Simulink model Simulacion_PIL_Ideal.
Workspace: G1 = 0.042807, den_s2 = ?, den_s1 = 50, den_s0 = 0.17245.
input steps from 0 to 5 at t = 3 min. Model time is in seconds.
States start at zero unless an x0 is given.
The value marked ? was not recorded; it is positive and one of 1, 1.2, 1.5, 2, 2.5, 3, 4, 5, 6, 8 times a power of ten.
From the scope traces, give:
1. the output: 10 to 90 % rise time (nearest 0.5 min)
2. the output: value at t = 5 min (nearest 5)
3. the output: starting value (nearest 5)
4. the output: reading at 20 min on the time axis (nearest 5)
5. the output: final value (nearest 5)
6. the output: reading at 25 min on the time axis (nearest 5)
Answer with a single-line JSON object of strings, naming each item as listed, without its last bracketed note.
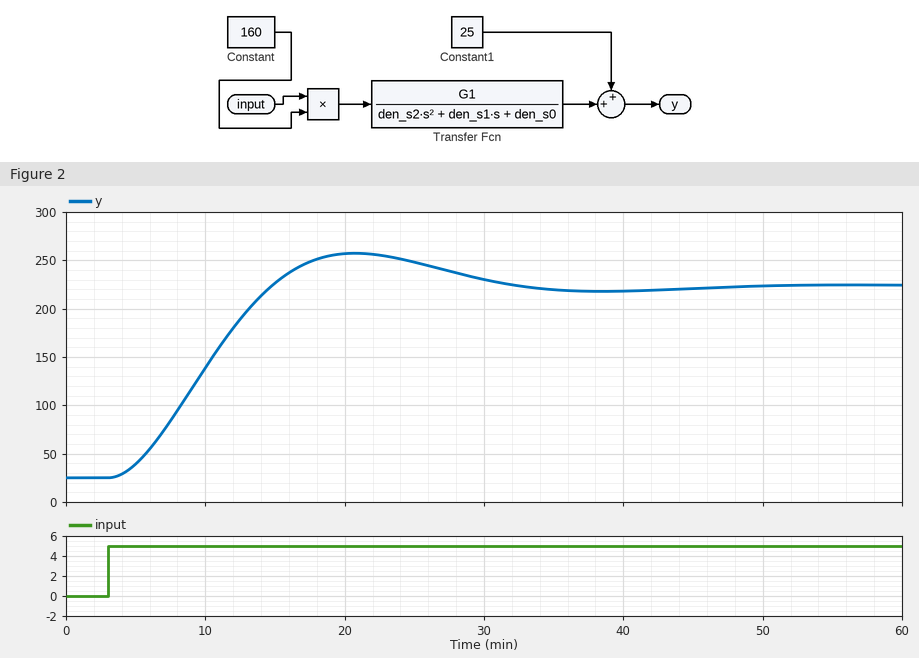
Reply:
{"the output: 10 to 90 % rise time": "8.0 min", "the output: value at t = 5 min": "40", "the output: starting value": "25", "the output: reading at 20 min on the time axis": "255", "the output: final value": "225", "the output: reading at 25 min on the time axis": "250"}
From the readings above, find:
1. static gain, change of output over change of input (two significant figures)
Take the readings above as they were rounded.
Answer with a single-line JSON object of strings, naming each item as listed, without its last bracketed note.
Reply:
{"static gain, change of output over change of input": "40"}
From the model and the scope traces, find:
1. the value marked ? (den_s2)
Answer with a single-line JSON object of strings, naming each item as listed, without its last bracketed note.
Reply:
{"the value marked ?": "15000"}
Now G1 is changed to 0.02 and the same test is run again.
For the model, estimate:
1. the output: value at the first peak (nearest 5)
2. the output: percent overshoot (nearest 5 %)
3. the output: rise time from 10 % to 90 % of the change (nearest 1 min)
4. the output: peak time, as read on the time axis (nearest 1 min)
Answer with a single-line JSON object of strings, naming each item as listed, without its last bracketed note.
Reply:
{"the output: value at the first peak": "135", "the output: percent overshoot": "15 %", "the output: rise time from 10 % to 90 % of the change": "8 min", "the output: peak time, as read on the time axis": "21 min"}
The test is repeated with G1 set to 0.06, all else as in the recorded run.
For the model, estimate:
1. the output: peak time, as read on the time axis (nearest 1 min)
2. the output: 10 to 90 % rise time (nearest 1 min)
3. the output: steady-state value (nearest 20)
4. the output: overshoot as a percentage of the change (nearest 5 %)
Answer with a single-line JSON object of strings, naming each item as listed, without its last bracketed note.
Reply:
{"the output: peak time, as read on the time axis": "21 min", "the output: 10 to 90 % rise time": "8 min", "the output: steady-state value": "300", "the output: overshoot as a percentage of the change": "15 %"}
